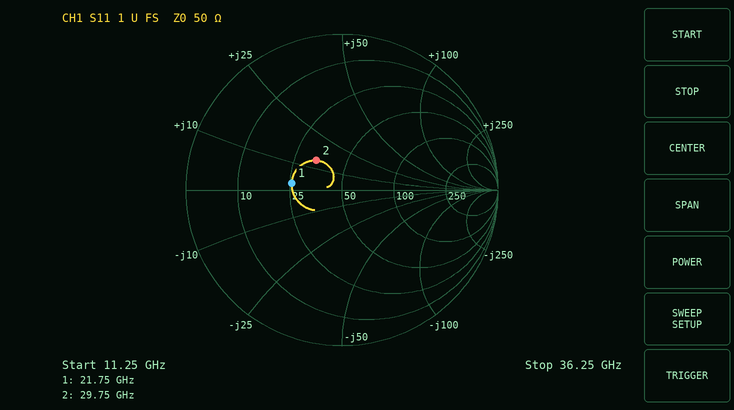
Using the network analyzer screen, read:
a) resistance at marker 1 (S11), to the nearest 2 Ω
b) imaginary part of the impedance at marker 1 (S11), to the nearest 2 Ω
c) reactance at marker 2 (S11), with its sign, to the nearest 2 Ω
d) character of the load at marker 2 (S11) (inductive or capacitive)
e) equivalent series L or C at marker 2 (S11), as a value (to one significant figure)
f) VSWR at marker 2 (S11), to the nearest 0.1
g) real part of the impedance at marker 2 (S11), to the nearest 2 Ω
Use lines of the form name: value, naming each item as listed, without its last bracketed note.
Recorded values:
resistance at marker 1 (S11), to the nearest 2 Ω: 26 Ω
imaginary part of the impedance at marker 1 (S11), to the nearest 2 Ω: +2 Ω
reactance at marker 2 (S11), with its sign, to the nearest 2 Ω: +14 Ω
character of the load at marker 2 (S11): inductive
equivalent series L or C at marker 2 (S11), as a value: 70 pH
VSWR at marker 2 (S11), to the nearest 0.1: 1.7
real part of the impedance at marker 2 (S11), to the nearest 2 Ω: 34 Ω
